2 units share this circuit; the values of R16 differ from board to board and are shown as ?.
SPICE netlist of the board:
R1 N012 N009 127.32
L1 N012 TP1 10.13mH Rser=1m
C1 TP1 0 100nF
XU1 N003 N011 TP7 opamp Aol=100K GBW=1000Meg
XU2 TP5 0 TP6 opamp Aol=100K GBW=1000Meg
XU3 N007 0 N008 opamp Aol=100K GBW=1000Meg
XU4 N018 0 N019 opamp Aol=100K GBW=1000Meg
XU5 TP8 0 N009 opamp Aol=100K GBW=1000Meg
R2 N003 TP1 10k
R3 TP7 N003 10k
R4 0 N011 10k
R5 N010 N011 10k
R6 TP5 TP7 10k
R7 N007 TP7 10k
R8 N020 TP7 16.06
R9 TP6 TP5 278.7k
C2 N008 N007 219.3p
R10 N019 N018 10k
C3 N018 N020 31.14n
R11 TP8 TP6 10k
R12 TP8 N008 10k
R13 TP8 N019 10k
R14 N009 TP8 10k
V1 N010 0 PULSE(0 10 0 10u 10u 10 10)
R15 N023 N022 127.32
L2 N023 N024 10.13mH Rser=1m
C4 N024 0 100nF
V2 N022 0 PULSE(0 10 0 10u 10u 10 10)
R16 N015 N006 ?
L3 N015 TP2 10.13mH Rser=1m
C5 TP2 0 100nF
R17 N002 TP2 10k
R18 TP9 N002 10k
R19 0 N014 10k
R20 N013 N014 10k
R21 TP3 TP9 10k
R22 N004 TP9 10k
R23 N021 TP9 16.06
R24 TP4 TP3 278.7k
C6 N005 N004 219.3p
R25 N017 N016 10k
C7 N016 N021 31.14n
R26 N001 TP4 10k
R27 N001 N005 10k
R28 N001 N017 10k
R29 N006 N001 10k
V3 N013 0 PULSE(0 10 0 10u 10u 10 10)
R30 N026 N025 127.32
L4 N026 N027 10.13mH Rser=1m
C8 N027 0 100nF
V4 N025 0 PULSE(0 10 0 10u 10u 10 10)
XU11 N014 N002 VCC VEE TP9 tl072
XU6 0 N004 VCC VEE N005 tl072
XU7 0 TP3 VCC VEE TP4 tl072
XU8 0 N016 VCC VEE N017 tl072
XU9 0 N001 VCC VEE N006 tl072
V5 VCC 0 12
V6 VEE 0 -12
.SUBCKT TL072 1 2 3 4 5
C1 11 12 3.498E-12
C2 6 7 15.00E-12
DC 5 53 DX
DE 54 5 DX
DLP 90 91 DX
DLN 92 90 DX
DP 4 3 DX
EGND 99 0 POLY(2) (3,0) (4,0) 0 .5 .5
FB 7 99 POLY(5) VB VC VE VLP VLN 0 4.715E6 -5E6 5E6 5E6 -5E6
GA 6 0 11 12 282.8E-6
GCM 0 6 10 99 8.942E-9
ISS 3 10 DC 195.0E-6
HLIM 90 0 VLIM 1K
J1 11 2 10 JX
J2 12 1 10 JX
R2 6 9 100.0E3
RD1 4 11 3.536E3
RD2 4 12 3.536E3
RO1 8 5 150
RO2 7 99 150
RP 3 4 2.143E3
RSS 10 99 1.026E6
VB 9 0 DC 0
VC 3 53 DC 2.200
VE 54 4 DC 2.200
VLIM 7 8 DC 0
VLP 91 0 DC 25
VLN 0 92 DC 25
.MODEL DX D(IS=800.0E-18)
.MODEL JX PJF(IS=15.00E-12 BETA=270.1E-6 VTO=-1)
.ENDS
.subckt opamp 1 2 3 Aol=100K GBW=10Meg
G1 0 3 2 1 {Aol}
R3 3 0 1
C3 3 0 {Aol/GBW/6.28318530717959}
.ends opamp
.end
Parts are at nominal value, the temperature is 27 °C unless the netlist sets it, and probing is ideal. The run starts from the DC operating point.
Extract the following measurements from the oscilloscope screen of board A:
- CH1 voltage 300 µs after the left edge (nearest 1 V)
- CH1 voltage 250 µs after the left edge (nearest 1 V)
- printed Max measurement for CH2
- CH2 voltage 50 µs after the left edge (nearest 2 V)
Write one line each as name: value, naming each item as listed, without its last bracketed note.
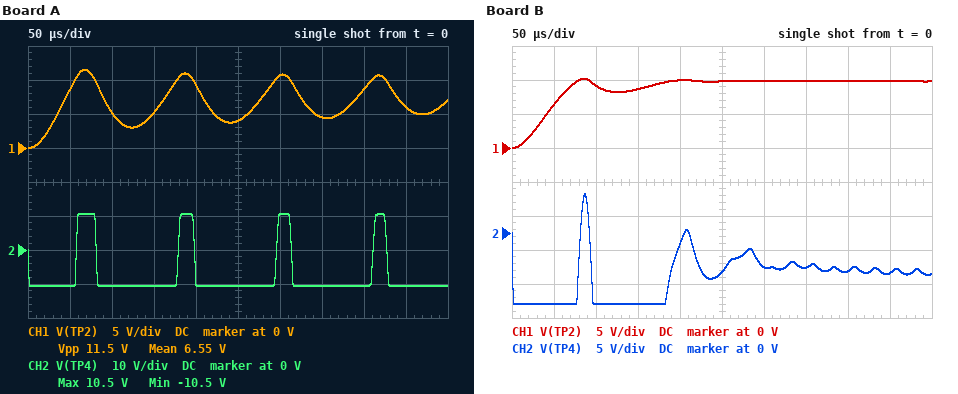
CH1 voltage 300 µs after the left edge: 11 V
CH1 voltage 250 µs after the left edge: 4 V
printed Max measurement for CH2: 10.5 V
CH2 voltage 50 µs after the left edge: -10 V
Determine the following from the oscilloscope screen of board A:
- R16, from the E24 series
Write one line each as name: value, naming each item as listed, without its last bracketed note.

R16, from the E24 series: 100 Ω
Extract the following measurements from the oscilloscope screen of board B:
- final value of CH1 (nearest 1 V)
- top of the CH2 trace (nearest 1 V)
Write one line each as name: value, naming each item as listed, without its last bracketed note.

final value of CH1: 10 V
top of the CH2 trace: 6 V
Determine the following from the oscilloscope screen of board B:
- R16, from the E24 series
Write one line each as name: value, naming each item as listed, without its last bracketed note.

R16, from the E24 series: 360 Ω
